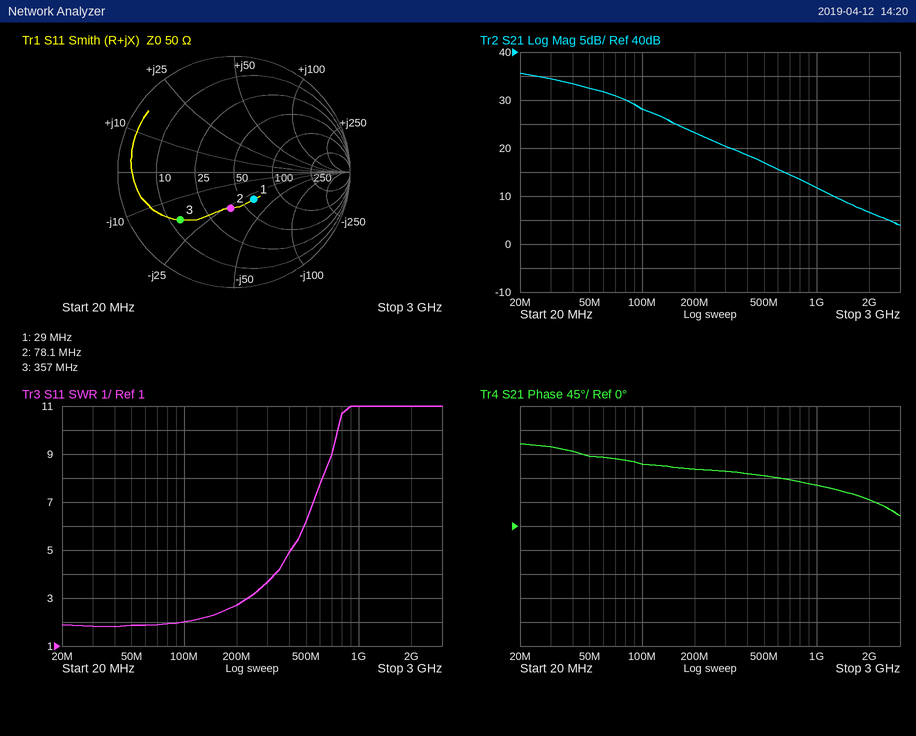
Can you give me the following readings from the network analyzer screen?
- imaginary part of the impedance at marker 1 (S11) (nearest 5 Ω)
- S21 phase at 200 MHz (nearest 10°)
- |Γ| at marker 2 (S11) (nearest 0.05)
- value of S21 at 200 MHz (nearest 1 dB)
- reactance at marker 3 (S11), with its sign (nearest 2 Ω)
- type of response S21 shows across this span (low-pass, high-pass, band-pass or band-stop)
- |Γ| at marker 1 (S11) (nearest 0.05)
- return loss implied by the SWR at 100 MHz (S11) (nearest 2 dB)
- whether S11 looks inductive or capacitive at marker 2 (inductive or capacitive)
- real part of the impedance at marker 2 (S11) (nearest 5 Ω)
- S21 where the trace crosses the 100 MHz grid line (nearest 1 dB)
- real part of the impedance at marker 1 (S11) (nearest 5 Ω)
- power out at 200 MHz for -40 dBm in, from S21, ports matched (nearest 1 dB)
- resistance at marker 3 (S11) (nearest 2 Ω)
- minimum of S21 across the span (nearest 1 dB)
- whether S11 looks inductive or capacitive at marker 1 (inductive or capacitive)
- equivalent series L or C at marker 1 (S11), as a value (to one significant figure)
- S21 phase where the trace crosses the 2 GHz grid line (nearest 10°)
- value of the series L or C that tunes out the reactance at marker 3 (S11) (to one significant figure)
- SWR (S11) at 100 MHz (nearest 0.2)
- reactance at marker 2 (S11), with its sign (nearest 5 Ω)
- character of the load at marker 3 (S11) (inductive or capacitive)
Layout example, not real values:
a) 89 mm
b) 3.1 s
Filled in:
a) -30 Ω
b) 110°
c) 0.30
d) 23 dB
e) -18 Ω
f) low-pass
g) 0.30
h) 10 dB
i) capacitive
j) 40 Ω
k) 28 dB
l) 60 Ω
m) -17 dBm
n) 14 Ω
o) 4 dB
p) capacitive
q) 200 pF
r) 50°
s) 8 nH
t) 2.0
u) -25 Ω
v) capacitive
